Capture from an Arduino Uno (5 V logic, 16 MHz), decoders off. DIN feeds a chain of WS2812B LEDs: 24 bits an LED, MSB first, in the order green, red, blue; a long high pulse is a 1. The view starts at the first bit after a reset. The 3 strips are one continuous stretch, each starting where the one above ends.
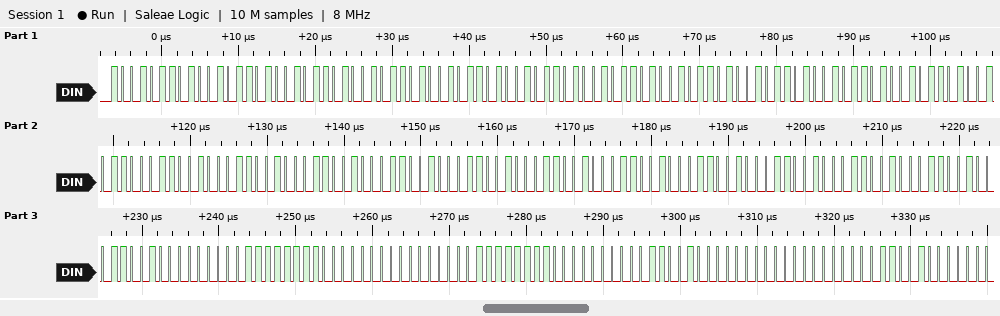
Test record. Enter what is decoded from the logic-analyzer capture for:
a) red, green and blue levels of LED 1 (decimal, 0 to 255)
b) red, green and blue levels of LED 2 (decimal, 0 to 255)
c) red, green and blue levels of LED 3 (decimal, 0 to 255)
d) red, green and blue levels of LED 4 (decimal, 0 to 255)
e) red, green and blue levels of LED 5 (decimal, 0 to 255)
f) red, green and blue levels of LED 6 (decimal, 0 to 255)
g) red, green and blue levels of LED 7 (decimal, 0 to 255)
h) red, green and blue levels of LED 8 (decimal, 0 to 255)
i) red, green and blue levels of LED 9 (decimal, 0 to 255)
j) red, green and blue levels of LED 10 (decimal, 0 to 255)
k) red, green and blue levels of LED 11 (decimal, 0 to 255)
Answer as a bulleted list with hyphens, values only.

- 150, 150, 150
- 150, 150, 150
- 150, 150, 150
- 150, 150, 150
- 50, 50, 50
- 50, 50, 50
- 50, 50, 50
- 50, 50, 50
- 255, 0, 0
- 255, 0, 0
- 0, 50, 0
